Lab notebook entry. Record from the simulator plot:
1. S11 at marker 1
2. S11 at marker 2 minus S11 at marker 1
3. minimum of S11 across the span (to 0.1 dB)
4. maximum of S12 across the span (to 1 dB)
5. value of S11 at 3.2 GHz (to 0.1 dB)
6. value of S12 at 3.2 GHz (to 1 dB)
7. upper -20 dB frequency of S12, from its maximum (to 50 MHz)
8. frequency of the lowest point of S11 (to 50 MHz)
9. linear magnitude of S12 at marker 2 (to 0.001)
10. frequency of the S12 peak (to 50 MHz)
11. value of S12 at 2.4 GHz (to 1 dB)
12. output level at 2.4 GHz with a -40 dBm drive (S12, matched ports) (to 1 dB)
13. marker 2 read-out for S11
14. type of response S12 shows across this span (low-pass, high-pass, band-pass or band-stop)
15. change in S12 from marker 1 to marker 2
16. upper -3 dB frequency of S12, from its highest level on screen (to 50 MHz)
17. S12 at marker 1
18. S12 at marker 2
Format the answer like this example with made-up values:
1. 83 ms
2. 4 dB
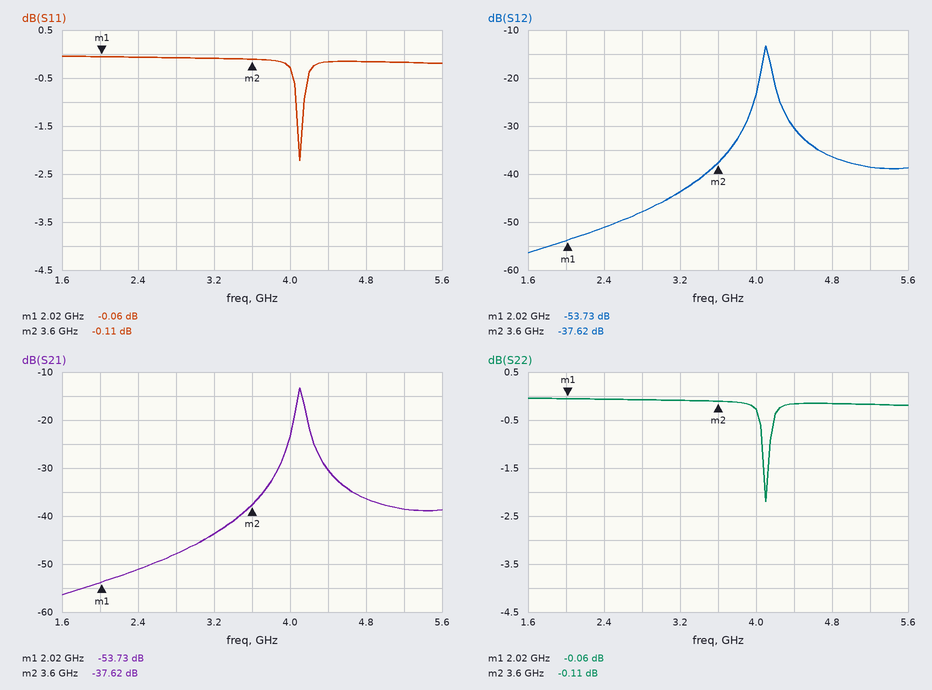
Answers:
1. -0.06 dB
2. -0.05 dB
3. -2.2 dB
4. -13 dB
5. -0.1 dB
6. -44 dB
7. 4.55 GHz
8. 4.10 GHz
9. 0.013
10. 4.10 GHz
11. -51 dB
12. -91 dBm
13. -0.11 dB
14. band-pass
15. 16.11 dB
16. 4.15 GHz
17. -53.73 dB
18. -37.62 dB
